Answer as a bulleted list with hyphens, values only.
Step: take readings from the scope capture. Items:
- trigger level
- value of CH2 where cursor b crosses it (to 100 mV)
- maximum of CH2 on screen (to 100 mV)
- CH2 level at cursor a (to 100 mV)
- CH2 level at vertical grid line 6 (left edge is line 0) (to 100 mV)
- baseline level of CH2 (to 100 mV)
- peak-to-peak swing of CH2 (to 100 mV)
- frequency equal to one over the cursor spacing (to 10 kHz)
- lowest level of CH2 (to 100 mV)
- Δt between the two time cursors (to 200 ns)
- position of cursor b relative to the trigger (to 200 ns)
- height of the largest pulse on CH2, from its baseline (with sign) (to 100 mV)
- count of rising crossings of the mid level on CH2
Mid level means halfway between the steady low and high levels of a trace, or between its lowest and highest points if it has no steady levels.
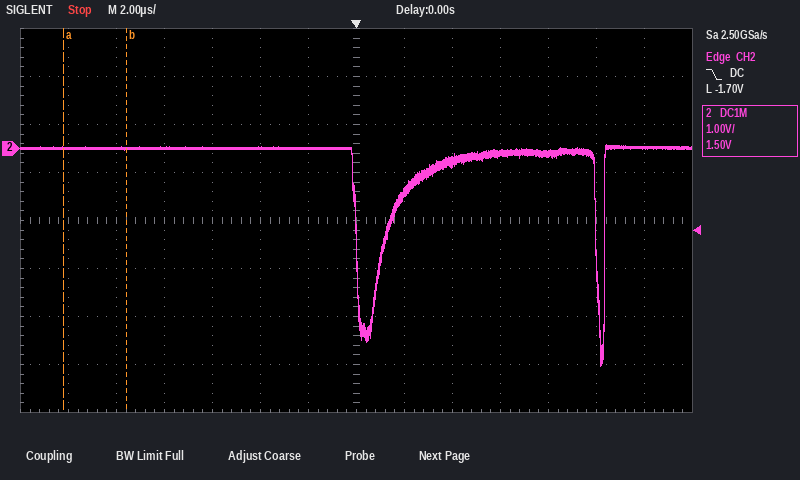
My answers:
- -1.70 V
- 0.0 V
- 100 mV
- 0.0 V
- 0.0 V
- 0.0 V
- 4.6 V
- 380 kHz
- -4.5 V
- 2.6 µs
- -9.6 µs
- -4.5 V
- 2
